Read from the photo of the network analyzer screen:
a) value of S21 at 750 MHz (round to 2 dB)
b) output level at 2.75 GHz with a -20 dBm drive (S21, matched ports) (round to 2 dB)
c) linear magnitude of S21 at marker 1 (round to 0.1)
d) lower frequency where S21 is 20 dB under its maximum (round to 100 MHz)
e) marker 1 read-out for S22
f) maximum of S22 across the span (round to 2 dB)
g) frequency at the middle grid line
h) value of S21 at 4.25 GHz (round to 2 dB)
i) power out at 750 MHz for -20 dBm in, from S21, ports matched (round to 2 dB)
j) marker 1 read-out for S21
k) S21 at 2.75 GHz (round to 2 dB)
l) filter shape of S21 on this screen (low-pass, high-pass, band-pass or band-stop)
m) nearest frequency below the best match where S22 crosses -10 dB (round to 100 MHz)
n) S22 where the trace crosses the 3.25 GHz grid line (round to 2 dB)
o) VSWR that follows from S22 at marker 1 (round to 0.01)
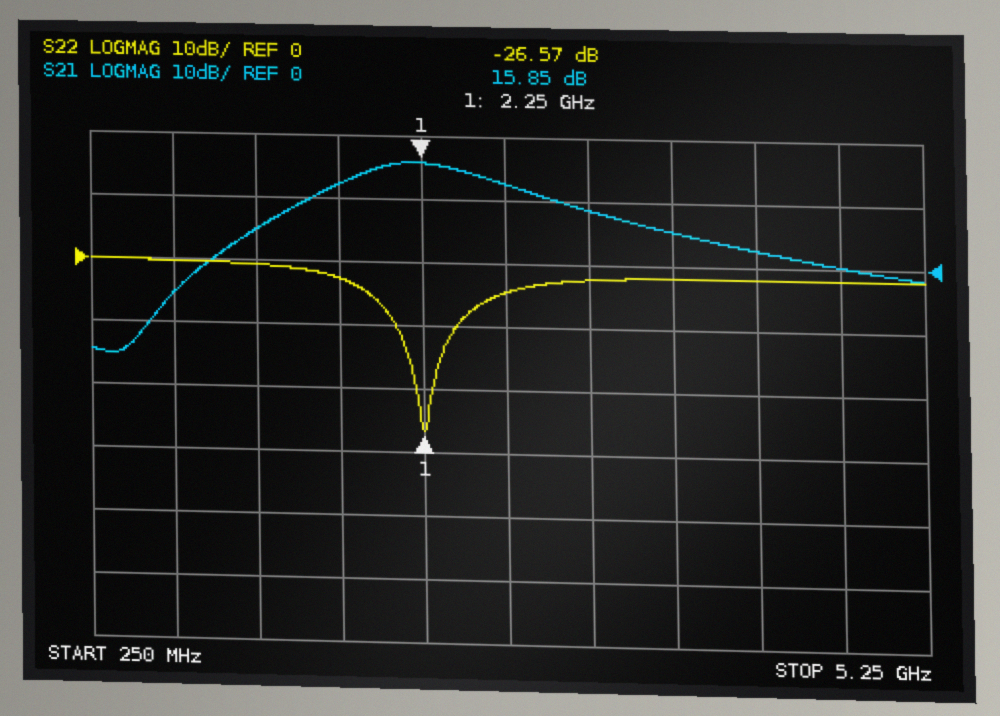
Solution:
-6 dB
-8 dBm
6.2
800 MHz
-26.57 dB
0 dB
2.75 GHz
2 dB
-26 dBm
15.85 dB
12 dB
band-pass
2.1 GHz
-2 dB
1.10
